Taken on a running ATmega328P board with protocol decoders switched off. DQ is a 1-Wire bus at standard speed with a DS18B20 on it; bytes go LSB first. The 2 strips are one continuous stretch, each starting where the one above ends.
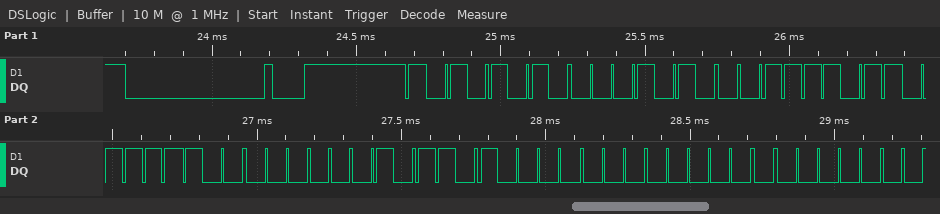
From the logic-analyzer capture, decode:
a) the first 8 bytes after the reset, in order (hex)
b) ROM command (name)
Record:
55 28 DE 3E 40 0B 00 00
Match ROM
